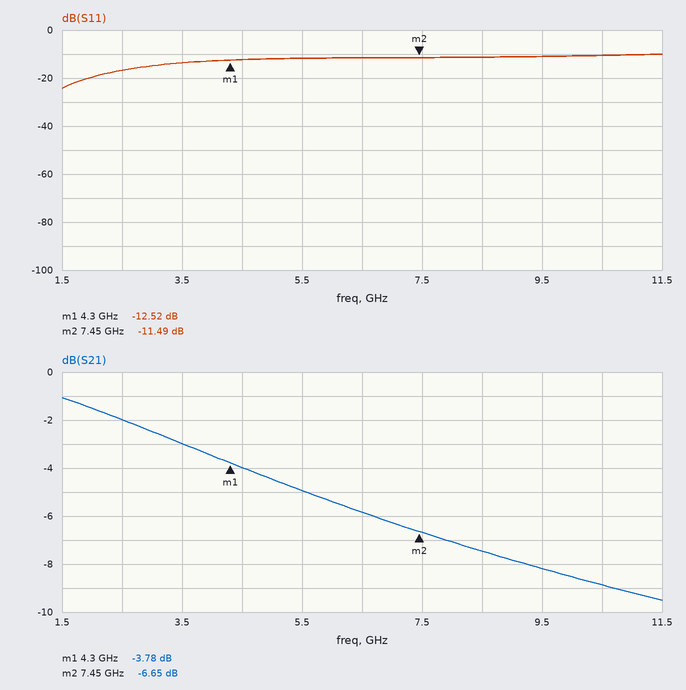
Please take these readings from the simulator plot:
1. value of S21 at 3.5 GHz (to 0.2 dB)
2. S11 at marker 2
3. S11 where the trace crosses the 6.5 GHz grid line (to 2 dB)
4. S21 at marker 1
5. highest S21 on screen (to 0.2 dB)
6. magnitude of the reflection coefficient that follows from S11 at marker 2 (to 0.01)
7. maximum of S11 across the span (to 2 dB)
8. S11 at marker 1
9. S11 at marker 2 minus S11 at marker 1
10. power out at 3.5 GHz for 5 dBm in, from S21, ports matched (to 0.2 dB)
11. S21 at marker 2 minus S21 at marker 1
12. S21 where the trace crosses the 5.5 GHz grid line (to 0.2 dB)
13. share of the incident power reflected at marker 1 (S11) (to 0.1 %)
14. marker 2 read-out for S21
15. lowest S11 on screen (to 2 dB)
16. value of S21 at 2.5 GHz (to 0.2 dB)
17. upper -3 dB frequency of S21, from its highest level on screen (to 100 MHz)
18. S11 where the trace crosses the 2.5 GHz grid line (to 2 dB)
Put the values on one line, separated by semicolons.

-3.0 dB; -11.49 dB; -12 dB; -3.78 dB; -1.0 dB; 0.27; -10 dB; -12.52 dB; 1.03 dB; 2.0 dBm; -2.87 dB; -5.0 dB; 5.6 %; -6.65 dB; -24 dB; -2.0 dB; 4.6 GHz; -16 dB
